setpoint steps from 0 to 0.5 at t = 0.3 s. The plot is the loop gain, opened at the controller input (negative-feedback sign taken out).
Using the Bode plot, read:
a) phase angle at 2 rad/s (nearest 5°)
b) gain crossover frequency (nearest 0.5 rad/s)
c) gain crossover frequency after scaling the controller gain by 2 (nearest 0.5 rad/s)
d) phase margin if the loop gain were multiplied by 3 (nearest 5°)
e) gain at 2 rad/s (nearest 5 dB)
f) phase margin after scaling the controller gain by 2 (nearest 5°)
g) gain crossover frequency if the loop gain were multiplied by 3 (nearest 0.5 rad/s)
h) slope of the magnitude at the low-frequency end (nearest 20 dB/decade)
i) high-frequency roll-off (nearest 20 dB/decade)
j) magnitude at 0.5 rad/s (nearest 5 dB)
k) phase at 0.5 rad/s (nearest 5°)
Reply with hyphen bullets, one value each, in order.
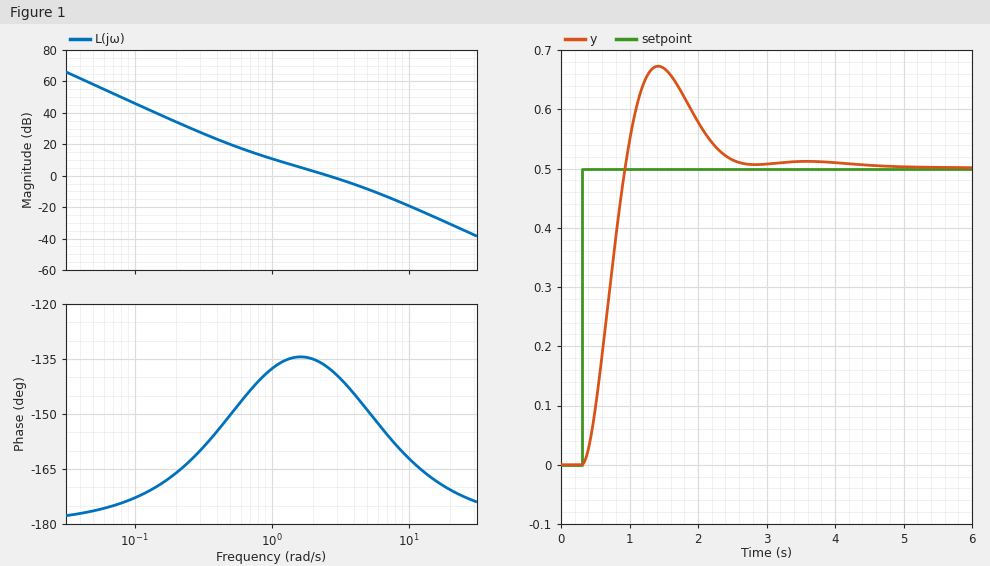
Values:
- -135°
- 2.5 rad/s
- 4.0 rad/s
- 30°
- 5 dB
- 35°
- 5.5 rad/s
- -40 dB/decade
- -40 dB/decade
- 20 dB
- -150°
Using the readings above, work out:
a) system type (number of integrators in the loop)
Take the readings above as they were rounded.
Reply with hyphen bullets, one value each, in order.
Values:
- 2
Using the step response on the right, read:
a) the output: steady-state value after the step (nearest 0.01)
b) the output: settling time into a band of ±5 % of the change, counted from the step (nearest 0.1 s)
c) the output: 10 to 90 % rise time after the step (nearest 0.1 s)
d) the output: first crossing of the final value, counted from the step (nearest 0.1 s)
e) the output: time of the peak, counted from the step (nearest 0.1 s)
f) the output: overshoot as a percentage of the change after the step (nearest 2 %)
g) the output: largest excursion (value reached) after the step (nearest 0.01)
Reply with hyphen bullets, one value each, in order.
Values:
- 0.50
- 2.1 s
- 0.4 s
- 0.6 s
- 1.1 s
- 34 %
- 0.67
